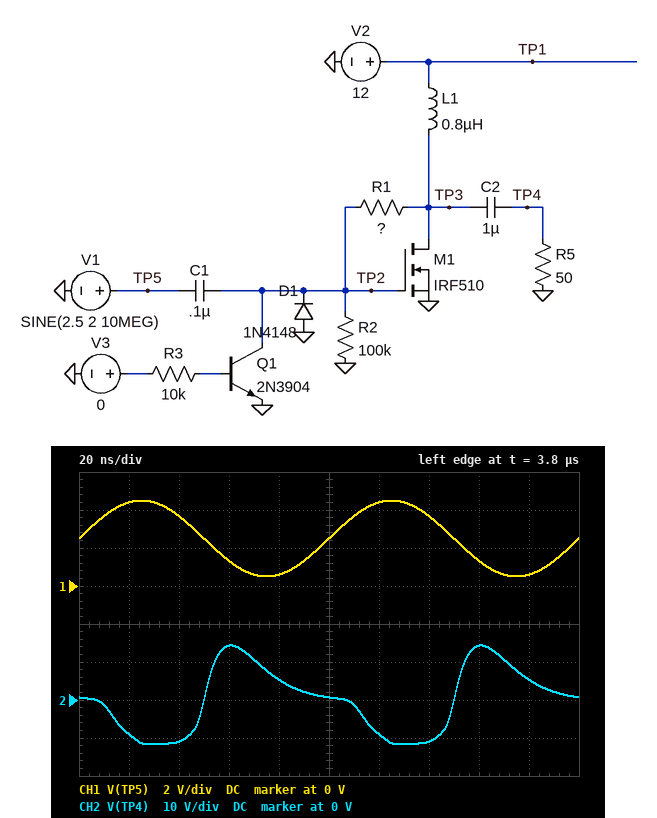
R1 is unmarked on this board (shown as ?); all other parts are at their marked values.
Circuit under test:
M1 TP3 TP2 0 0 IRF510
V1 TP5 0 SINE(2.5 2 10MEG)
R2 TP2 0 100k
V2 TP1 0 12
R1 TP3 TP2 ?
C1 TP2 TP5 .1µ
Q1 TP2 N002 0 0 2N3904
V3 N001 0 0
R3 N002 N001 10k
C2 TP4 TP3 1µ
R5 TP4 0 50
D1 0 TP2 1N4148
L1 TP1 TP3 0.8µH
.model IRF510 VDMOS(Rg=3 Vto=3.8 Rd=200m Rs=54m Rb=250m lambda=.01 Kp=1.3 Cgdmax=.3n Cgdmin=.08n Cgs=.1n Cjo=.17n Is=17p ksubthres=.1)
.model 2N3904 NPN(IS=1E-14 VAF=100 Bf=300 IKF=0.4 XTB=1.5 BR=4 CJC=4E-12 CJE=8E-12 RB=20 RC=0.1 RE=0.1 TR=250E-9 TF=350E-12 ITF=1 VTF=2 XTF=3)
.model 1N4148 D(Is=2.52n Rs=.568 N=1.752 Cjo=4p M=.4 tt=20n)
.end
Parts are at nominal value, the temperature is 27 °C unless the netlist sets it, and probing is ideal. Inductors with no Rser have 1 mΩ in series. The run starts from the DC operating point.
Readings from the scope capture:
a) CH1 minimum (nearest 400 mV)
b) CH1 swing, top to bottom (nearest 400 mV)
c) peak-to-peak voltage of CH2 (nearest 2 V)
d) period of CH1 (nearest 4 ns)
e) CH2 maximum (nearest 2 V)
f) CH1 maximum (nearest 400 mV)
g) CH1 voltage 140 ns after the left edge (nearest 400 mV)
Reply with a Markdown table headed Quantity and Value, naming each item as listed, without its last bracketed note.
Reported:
| Quantity | Value |
|---|---|
| CH1 minimum | 400 mV |
| CH1 swing, top to bottom | 4.0 V |
| peak-to-peak voltage of CH2 | 26 V |
| period of CH1 | 100 ns |
| CH2 maximum | 14 V |
| CH1 maximum | 4.4 V |
| CH1 voltage 140 ns after the left edge | 3.6 V |
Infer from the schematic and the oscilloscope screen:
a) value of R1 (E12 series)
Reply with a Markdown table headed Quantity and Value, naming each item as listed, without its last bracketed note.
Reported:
| Quantity | Value |
|---|---|
| value of R1 | 270 kΩ |
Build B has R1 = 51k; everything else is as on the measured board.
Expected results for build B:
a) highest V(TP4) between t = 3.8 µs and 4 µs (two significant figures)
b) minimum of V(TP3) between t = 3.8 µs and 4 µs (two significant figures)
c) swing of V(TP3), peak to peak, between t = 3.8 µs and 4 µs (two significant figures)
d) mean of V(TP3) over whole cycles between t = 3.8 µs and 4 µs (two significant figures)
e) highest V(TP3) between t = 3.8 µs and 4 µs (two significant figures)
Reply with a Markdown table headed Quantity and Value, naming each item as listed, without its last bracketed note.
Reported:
| Quantity | Value |
|---|---|
| highest V(TP4) between t = 3.8 µs and 4 µs | 30 V |
| minimum of V(TP3) between t = 3.8 µs and 4 µs | 2.2 V |
| swing of V(TP3), peak to peak, between t = 3.8 µs and 4 µs | 40 V |
| mean of V(TP3) over whole cycles between t = 3.8 µs and 4 µs | 12 V |
| highest V(TP3) between t = 3.8 µs and 4 µs | 42 V |
